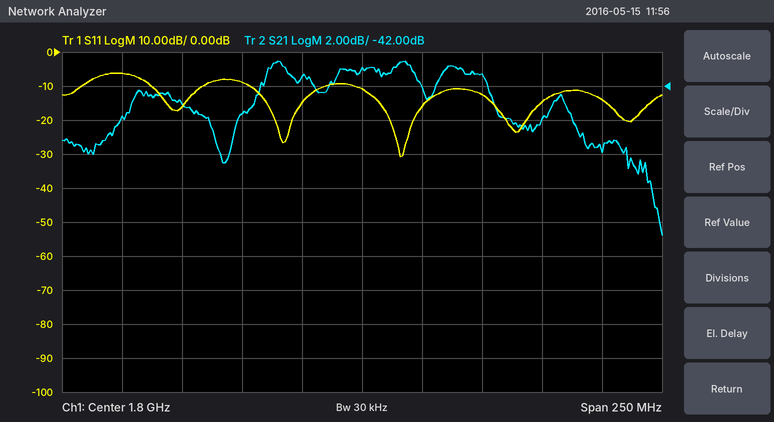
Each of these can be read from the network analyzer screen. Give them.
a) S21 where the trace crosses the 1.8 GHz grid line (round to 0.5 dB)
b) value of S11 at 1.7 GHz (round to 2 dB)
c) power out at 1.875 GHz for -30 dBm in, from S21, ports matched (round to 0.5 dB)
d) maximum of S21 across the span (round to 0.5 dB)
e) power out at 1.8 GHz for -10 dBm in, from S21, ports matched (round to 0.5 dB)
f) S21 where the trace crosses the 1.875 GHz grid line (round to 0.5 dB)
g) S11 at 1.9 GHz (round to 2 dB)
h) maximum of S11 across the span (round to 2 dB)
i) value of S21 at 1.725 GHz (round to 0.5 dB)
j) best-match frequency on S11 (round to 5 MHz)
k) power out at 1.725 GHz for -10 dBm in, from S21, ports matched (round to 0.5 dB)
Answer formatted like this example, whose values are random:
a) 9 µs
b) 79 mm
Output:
a) -41.0 dB
b) -6 dB
c) -74.0 dBm
d) -40.5 dB
e) -51.0 dBm
f) -44.0 dB
g) -14 dB
h) -6 dB
i) -43.0 dB
j) 1.815 GHz
k) -53.0 dBm
